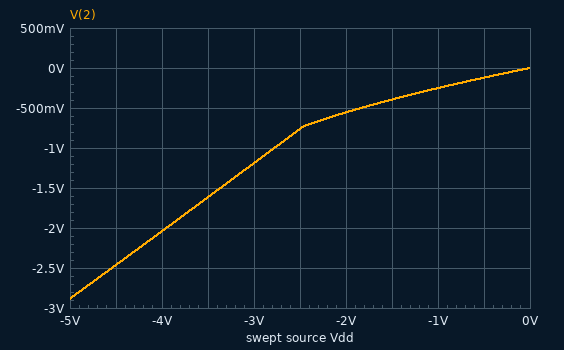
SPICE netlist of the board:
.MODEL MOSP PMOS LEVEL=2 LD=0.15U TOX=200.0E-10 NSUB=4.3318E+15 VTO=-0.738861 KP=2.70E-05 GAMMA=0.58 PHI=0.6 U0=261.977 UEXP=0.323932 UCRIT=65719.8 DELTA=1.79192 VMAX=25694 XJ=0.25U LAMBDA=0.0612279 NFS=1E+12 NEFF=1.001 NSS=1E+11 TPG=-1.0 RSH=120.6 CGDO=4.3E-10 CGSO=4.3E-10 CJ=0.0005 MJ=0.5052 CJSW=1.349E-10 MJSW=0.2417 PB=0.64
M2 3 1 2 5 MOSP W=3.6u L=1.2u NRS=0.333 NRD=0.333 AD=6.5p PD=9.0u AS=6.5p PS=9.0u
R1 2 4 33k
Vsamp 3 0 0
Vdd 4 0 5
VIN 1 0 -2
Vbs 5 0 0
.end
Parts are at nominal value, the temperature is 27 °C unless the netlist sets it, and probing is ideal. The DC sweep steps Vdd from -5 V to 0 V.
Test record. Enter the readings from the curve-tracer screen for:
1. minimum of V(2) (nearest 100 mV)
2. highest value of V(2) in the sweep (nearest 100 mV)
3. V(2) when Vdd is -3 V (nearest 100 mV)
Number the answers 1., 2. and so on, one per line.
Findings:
1. -2.9 V
2. 0 V
3. -1.2 V
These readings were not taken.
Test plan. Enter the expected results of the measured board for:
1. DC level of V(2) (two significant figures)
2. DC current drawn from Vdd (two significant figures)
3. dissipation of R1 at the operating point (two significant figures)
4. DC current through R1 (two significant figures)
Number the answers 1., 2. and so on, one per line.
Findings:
1. 590 mV
2. 130 µA
3. 590 µW
4. 130 µA
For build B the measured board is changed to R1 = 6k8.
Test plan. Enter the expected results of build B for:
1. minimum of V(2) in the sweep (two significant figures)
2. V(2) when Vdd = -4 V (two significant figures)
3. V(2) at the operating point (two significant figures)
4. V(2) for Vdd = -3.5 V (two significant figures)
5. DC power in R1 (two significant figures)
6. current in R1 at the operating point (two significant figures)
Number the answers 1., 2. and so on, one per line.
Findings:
1. -4.5 V
2. -3.5 V
3. 670 mV
4. -3.1 V
5. 2.8 mW
6. 640 µA
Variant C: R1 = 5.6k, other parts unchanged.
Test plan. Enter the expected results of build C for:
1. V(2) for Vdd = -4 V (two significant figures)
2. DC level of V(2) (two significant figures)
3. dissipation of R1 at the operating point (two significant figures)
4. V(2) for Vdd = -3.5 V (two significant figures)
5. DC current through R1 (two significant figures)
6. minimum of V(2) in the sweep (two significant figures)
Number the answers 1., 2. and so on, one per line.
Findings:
1. -3.6 V
2. 680 mV
3. 3.3 mW
4. -3.1 V
5. 770 µA
6. -4.6 V
